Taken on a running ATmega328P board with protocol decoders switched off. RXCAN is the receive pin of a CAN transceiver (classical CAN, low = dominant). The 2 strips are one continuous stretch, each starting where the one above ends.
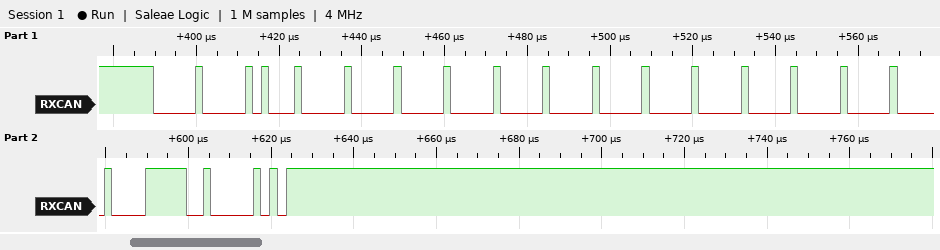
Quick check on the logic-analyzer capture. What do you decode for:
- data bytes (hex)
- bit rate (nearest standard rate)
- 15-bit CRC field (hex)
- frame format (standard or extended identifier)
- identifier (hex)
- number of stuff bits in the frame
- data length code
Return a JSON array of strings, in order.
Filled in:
["00 00 00 00 00 00 00 00", "500 kbit/s", "0x1F40", "standard", "0x001", "17", "8"]
